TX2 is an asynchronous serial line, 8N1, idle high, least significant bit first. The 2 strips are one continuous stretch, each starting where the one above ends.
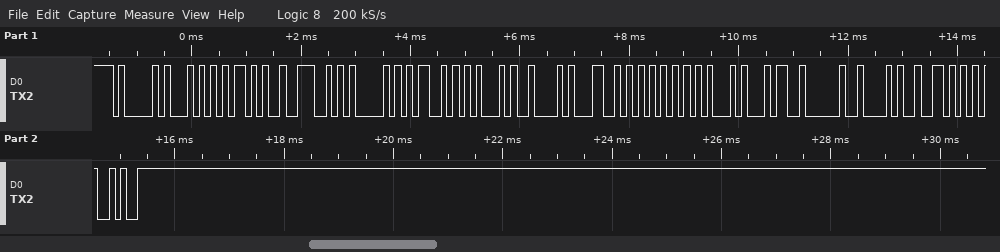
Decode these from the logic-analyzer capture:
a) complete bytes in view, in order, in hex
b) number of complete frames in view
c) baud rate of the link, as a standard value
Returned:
41 54 2B 4E 41 4D 45 42 4C 55 45 34 20 28 56 29
16
9600 baud
